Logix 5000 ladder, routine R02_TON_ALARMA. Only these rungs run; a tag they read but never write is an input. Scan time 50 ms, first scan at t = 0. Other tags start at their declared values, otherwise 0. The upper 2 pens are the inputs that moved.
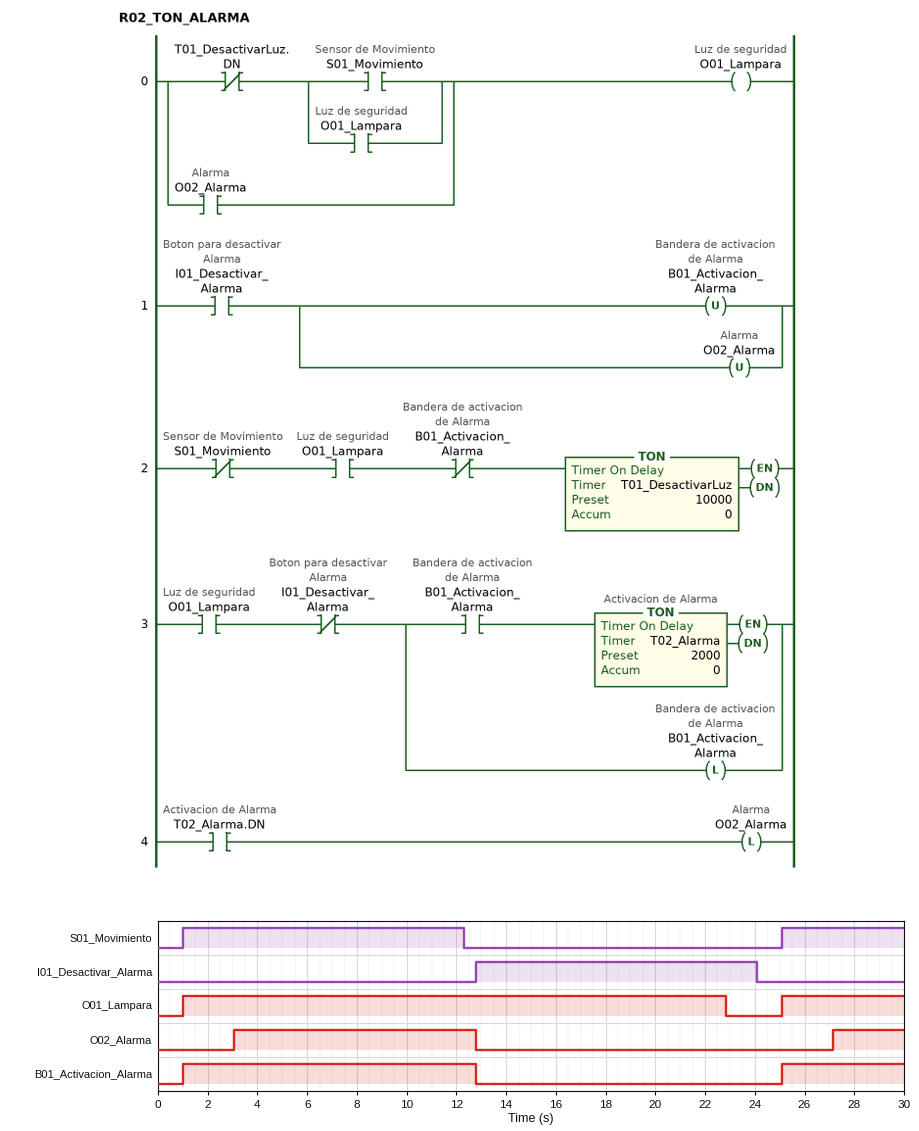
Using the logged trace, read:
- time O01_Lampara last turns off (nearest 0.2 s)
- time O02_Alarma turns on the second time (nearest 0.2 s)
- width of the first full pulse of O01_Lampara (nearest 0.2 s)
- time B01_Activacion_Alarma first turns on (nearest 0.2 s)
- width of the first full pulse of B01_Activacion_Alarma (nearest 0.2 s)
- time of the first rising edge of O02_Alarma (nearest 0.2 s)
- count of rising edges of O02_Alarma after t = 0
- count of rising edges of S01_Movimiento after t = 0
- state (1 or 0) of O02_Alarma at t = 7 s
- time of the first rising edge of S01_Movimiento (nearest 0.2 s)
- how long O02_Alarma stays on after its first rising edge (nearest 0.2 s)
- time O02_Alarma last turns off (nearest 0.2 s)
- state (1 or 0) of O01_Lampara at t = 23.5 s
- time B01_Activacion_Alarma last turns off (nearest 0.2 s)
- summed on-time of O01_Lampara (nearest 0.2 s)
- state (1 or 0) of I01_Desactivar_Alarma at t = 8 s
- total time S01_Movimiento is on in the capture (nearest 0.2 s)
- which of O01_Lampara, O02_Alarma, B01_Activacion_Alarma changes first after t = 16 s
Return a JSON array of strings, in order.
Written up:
["22.8 s", "27.2 s", "21.8 s", "1.0 s", "11.8 s", "3.0 s", "2", "2", "1", "1.0 s", "9.8 s", "12.8 s", "0", "12.8 s", "26.8 s", "0", "16.2 s", "O01_Lampara"]
